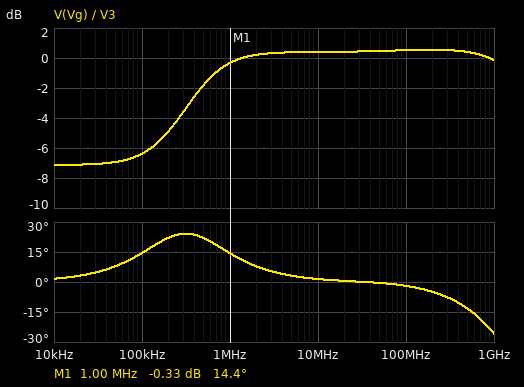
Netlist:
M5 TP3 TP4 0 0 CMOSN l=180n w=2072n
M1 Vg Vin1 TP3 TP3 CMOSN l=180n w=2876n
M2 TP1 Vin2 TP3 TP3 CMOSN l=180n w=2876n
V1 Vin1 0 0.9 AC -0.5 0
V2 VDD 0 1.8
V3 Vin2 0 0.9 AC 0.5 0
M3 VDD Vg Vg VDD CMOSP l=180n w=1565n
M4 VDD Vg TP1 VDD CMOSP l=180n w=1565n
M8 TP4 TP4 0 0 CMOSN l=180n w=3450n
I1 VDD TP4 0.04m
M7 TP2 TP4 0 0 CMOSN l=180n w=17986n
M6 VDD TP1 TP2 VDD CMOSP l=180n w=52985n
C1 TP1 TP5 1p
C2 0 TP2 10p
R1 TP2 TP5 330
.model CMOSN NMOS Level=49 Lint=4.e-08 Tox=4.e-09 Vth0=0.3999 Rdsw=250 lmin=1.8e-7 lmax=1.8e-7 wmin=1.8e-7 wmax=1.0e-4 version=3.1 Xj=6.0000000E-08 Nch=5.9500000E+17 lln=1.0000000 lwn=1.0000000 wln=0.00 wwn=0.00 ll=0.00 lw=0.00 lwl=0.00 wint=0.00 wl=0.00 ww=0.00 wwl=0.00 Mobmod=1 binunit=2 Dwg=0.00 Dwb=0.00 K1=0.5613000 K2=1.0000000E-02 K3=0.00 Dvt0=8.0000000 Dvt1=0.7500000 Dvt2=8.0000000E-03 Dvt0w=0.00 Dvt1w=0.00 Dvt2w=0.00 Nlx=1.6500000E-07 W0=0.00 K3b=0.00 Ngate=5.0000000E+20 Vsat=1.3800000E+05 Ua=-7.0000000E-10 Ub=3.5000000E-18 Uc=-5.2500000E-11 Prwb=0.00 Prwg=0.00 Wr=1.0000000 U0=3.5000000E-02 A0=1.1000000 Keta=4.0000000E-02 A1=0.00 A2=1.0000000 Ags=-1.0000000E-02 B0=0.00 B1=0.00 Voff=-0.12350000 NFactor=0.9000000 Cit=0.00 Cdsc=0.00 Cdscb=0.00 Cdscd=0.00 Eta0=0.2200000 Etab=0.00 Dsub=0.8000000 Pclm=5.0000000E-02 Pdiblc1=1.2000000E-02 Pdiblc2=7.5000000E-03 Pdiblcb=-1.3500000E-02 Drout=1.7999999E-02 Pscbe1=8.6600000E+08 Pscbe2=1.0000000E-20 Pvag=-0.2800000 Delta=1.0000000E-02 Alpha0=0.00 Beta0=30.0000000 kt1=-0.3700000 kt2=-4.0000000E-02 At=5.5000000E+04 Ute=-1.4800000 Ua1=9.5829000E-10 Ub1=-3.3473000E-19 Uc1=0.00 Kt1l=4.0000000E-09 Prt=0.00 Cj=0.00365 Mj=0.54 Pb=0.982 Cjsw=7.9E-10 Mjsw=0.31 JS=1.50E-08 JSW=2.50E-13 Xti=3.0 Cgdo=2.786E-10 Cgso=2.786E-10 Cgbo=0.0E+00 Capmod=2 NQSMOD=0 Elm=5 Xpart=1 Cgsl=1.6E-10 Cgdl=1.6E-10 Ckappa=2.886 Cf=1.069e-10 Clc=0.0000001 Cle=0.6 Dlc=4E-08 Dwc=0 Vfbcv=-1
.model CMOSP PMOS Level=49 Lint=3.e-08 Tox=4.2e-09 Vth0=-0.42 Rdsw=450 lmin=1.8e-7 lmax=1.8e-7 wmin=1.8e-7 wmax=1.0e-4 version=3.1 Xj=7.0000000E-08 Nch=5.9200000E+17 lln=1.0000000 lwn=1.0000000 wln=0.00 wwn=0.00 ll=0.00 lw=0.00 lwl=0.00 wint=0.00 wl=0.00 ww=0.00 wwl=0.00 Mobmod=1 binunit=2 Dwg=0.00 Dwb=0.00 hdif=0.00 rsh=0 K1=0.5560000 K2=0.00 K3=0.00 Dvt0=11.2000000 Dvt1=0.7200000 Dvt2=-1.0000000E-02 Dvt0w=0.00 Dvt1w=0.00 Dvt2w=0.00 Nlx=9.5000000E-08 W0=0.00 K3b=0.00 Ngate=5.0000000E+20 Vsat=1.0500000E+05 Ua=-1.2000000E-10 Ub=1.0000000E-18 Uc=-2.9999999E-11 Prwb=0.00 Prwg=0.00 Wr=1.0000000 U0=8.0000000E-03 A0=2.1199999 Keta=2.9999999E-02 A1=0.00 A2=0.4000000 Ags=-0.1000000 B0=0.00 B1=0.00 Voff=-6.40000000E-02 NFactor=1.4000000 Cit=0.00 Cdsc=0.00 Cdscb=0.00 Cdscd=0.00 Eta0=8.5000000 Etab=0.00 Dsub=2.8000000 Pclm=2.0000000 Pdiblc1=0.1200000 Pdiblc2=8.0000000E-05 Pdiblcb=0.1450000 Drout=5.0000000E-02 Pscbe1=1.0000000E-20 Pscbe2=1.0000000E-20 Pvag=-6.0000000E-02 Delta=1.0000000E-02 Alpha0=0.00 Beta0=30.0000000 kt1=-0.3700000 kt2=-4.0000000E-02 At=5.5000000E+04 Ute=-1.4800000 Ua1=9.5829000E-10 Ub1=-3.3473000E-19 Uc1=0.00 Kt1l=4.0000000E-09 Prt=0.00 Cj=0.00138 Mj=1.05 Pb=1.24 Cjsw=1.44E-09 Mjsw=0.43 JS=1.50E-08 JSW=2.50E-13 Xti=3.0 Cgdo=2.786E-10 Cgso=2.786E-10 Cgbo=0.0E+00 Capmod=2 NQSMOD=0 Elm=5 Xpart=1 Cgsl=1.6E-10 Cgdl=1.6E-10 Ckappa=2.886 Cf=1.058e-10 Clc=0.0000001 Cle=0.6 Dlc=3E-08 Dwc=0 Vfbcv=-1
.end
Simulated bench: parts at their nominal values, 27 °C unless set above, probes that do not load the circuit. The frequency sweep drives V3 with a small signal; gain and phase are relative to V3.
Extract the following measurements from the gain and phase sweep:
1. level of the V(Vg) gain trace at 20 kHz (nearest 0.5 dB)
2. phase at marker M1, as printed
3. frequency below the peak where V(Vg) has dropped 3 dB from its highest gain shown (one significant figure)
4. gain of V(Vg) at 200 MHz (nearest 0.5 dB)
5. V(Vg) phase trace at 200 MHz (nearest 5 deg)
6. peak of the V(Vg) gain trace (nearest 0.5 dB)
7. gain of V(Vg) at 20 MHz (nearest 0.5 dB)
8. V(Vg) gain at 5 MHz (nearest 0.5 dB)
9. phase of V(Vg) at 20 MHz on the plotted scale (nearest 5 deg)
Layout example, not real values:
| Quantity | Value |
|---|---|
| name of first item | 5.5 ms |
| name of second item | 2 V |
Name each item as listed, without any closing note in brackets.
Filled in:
| Quantity | Value |
|---|---|
| level of the V(Vg) gain trace at 20 kHz | -7.0 dB |
| phase at marker M1, as printed | 14.4 deg |
| frequency below the peak where V(Vg) has dropped 3 dB from its highest gain shown | 400 kHz |
| gain of V(Vg) at 200 MHz | 0.5 dB |
| V(Vg) phase trace at 200 MHz | -5 deg |
| peak of the V(Vg) gain trace | 0.5 dB |
| gain of V(Vg) at 20 MHz | 0.5 dB |
| V(Vg) gain at 5 MHz | 0.5 dB |
| phase of V(Vg) at 20 MHz on the plotted scale | 0 deg |
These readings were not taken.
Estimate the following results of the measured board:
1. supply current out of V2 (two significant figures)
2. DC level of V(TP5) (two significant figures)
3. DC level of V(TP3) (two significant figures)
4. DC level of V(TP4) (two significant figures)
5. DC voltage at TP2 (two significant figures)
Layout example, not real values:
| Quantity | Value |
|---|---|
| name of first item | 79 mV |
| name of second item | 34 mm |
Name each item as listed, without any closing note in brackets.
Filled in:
| Quantity | Value |
|---|---|
| supply current out of V2 | 520 µA |
| DC level of V(TP5) | 1.3 V |
| DC level of V(TP3) | 510 mV |
| DC level of V(TP4) | 480 mV |
| DC voltage at TP2 | 1.3 V |
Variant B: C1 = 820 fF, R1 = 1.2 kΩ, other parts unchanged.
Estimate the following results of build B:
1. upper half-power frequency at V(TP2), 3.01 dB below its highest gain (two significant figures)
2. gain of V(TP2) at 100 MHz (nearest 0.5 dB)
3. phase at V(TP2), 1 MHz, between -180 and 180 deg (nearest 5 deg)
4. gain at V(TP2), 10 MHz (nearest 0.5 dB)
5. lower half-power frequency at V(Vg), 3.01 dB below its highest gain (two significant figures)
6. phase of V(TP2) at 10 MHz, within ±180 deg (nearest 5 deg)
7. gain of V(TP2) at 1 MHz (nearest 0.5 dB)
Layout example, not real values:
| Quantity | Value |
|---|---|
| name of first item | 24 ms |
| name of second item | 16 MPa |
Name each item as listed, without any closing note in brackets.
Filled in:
| Quantity | Value |
|---|---|
| upper half-power frequency at V(TP2), 3.01 dB below its highest gain | 580 kHz |
| gain of V(TP2) at 100 MHz | -9.0 dB |
| phase at V(TP2), 1 MHz, between -180 and 180 deg | -60 deg |
| gain at V(TP2), 10 MHz | 13.5 dB |
| lower half-power frequency at V(Vg), 3.01 dB below its highest gain | 480 kHz |
| phase of V(TP2) at 10 MHz, within ±180 deg | -90 deg |
| gain of V(TP2) at 1 MHz | 32.5 dB |
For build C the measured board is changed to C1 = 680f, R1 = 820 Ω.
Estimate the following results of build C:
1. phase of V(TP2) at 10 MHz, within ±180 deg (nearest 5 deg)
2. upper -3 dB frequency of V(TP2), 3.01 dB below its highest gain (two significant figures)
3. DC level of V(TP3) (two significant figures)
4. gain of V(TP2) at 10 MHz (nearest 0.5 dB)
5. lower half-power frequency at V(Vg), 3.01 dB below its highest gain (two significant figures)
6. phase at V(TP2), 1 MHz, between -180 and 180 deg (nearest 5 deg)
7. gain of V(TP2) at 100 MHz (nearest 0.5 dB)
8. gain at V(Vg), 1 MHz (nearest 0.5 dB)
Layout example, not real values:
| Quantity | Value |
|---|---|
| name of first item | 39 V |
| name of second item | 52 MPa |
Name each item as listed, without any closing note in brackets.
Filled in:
| Quantity | Value |
|---|---|
| phase of V(TP2) at 10 MHz, within ±180 deg | -90 deg |
| upper -3 dB frequency of V(TP2), 3.01 dB below its highest gain | 690 kHz |
| DC level of V(TP3) | 510 mV |
| gain of V(TP2) at 10 MHz | 15.0 dB |
| lower half-power frequency at V(Vg), 3.01 dB below its highest gain | 580 kHz |
| phase at V(TP2), 1 MHz, between -180 and 180 deg | -55 deg |
| gain of V(TP2) at 100 MHz | -8.5 dB |
| gain at V(Vg), 1 MHz | -1.0 dB |
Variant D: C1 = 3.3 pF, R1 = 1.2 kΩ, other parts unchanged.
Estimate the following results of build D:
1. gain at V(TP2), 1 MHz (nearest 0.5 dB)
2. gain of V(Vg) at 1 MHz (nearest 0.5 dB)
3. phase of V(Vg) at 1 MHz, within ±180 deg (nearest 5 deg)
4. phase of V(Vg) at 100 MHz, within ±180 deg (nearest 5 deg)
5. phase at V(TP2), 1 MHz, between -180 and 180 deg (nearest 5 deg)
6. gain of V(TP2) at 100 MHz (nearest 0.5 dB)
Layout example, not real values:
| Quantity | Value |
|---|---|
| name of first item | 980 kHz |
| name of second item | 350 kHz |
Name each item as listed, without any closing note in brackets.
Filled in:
| Quantity | Value |
|---|---|
| gain at V(TP2), 1 MHz | 22.0 dB |
| gain of V(Vg) at 1 MHz | 0.5 dB |
| phase of V(Vg) at 1 MHz, within ±180 deg | 5 deg |
| phase of V(Vg) at 100 MHz, within ±180 deg | -5 deg |
| phase at V(TP2), 1 MHz, between -180 and 180 deg | -80 deg |
| gain of V(TP2) at 100 MHz | -14.5 dB |
